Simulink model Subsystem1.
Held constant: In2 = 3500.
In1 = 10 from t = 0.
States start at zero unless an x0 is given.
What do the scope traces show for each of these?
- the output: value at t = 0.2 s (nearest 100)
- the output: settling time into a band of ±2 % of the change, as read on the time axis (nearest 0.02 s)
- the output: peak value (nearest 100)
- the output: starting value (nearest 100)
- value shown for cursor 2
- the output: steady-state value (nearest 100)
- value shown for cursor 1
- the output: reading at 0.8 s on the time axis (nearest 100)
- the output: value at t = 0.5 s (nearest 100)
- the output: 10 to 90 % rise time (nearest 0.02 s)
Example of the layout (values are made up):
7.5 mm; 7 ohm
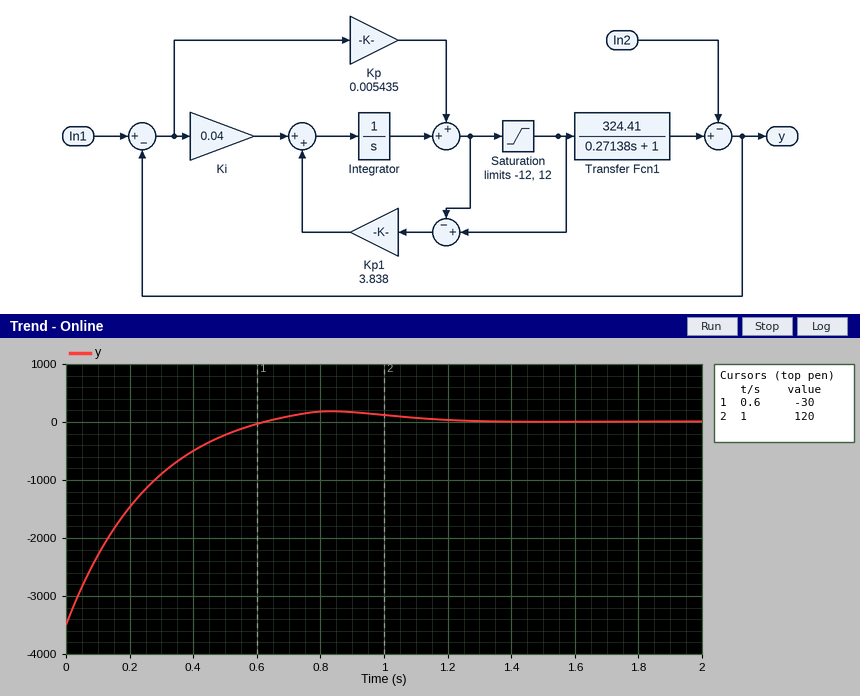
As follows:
-1500; 1.08 s; 200; -3500; 120; 0; -30; 200; -200; 0.42 s
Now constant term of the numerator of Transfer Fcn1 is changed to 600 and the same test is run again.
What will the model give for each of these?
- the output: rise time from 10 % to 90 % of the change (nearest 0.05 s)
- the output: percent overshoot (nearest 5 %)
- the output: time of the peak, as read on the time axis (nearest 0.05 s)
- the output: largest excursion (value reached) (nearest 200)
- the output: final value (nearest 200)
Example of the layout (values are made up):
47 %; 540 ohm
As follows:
0.15 s; 10 %; 0.30 s; 400; 0
